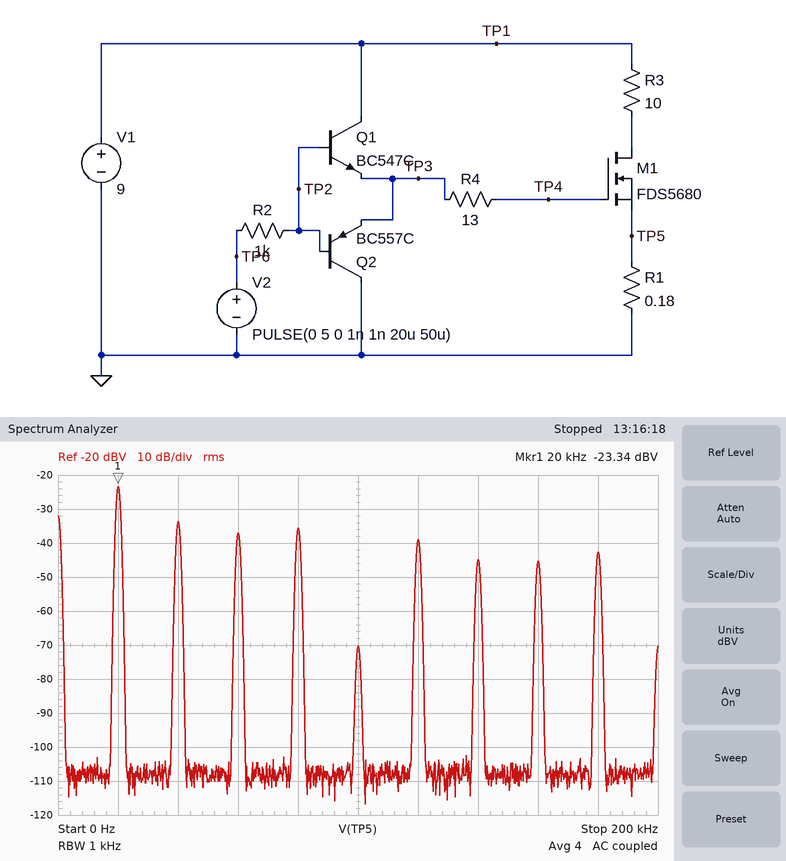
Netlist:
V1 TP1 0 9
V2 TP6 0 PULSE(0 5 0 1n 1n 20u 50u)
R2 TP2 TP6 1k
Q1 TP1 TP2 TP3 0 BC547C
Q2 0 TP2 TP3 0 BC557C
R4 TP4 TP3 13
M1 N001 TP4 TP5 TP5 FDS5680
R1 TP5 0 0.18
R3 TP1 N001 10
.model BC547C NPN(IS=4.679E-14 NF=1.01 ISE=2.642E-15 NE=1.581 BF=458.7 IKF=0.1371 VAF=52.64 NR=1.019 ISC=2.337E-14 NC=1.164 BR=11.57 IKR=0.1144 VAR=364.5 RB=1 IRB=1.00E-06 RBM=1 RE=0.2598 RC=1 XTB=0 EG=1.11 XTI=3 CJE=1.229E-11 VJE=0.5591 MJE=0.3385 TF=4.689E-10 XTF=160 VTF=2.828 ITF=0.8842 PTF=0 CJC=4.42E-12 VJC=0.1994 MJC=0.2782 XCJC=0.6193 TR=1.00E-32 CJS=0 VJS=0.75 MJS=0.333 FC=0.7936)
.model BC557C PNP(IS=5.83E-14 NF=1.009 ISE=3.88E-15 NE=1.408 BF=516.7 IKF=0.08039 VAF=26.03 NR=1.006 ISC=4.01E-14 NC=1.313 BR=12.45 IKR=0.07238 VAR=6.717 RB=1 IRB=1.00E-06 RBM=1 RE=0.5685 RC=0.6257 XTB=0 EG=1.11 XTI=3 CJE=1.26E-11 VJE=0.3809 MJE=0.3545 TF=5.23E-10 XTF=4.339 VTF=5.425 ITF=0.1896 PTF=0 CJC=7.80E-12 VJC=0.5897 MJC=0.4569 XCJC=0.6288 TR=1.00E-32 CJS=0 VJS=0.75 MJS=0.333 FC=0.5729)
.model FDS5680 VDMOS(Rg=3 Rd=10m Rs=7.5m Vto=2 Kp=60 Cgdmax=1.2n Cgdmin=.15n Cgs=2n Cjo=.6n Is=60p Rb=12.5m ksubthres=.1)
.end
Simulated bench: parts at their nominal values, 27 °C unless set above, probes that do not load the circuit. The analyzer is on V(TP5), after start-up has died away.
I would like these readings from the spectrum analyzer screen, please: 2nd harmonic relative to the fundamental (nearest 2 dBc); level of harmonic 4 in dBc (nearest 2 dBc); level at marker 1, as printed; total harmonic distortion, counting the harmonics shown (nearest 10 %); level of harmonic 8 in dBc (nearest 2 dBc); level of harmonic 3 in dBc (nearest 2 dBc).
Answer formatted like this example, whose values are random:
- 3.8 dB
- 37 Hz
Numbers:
- -10 dBc
- -12 dBc
- -23.34 dBV
- 50 %
- -22 dBc
- -14 dBc
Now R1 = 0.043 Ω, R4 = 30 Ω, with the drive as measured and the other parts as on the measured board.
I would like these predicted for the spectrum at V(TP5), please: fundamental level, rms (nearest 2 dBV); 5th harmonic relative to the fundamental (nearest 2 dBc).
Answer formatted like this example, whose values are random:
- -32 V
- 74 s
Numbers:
- -36 dBV
- -42 dBc
